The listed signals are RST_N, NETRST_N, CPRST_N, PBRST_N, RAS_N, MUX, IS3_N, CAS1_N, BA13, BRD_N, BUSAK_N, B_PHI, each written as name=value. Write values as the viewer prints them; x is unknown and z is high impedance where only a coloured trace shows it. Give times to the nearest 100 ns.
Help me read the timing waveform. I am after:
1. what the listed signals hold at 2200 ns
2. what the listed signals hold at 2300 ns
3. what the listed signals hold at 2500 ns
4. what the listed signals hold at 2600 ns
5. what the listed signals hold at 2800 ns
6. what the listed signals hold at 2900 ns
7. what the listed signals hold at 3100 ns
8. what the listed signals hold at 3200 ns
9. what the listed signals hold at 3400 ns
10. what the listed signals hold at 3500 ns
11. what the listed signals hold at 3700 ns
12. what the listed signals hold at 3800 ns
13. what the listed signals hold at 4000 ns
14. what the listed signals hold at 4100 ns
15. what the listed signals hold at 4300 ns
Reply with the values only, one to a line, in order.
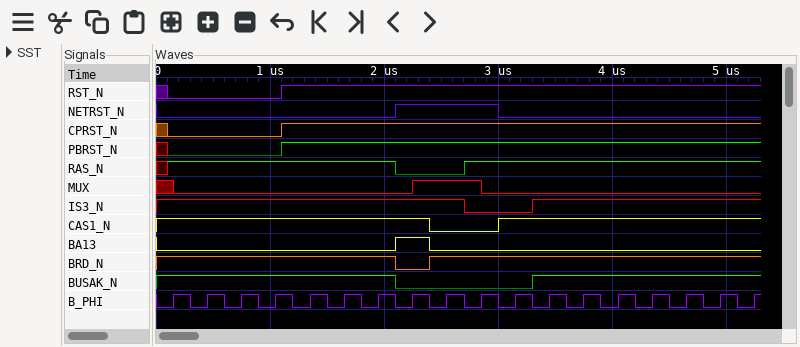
RST_N=1, NETRST_N=1, CPRST_N=1, PBRST_N=1, RAS_N=0, MUX=0, IS3_N=1, CAS1_N=1, BA13=1, BRD_N=0, BUSAK_N=0, B_PHI=0
RST_N=1, NETRST_N=1, CPRST_N=1, PBRST_N=1, RAS_N=0, MUX=1, IS3_N=1, CAS1_N=1, BA13=1, BRD_N=0, BUSAK_N=0, B_PHI=1
RST_N=1, NETRST_N=1, CPRST_N=1, PBRST_N=1, RAS_N=0, MUX=1, IS3_N=1, CAS1_N=0, BA13=0, BRD_N=1, BUSAK_N=0, B_PHI=0
RST_N=1, NETRST_N=1, CPRST_N=1, PBRST_N=1, RAS_N=0, MUX=1, IS3_N=1, CAS1_N=0, BA13=0, BRD_N=1, BUSAK_N=0, B_PHI=1
RST_N=1, NETRST_N=1, CPRST_N=1, PBRST_N=1, RAS_N=1, MUX=1, IS3_N=0, CAS1_N=0, BA13=0, BRD_N=1, BUSAK_N=0, B_PHI=0
RST_N=1, NETRST_N=1, CPRST_N=1, PBRST_N=1, RAS_N=1, MUX=0, IS3_N=0, CAS1_N=0, BA13=0, BRD_N=1, BUSAK_N=0, B_PHI=1
RST_N=1, NETRST_N=0, CPRST_N=1, PBRST_N=1, RAS_N=1, MUX=0, IS3_N=0, CAS1_N=1, BA13=0, BRD_N=1, BUSAK_N=0, B_PHI=0
RST_N=1, NETRST_N=0, CPRST_N=1, PBRST_N=1, RAS_N=1, MUX=0, IS3_N=0, CAS1_N=1, BA13=0, BRD_N=1, BUSAK_N=0, B_PHI=1
RST_N=1, NETRST_N=0, CPRST_N=1, PBRST_N=1, RAS_N=1, MUX=0, IS3_N=1, CAS1_N=1, BA13=0, BRD_N=1, BUSAK_N=1, B_PHI=0
RST_N=1, NETRST_N=0, CPRST_N=1, PBRST_N=1, RAS_N=1, MUX=0, IS3_N=1, CAS1_N=1, BA13=0, BRD_N=1, BUSAK_N=1, B_PHI=1
RST_N=1, NETRST_N=0, CPRST_N=1, PBRST_N=1, RAS_N=1, MUX=0, IS3_N=1, CAS1_N=1, BA13=0, BRD_N=1, BUSAK_N=1, B_PHI=0
RST_N=1, NETRST_N=0, CPRST_N=1, PBRST_N=1, RAS_N=1, MUX=0, IS3_N=1, CAS1_N=1, BA13=0, BRD_N=1, BUSAK_N=1, B_PHI=1
RST_N=1, NETRST_N=0, CPRST_N=1, PBRST_N=1, RAS_N=1, MUX=0, IS3_N=1, CAS1_N=1, BA13=0, BRD_N=1, BUSAK_N=1, B_PHI=0
RST_N=1, NETRST_N=0, CPRST_N=1, PBRST_N=1, RAS_N=1, MUX=0, IS3_N=1, CAS1_N=1, BA13=0, BRD_N=1, BUSAK_N=1, B_PHI=1
RST_N=1, NETRST_N=0, CPRST_N=1, PBRST_N=1, RAS_N=1, MUX=0, IS3_N=1, CAS1_N=1, BA13=0, BRD_N=1, BUSAK_N=1, B_PHI=0
